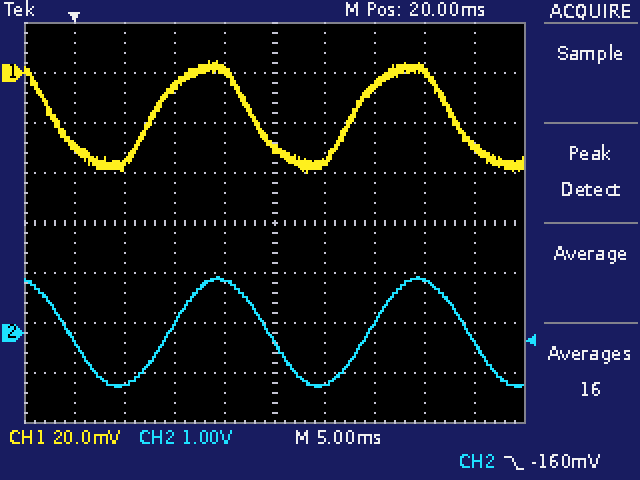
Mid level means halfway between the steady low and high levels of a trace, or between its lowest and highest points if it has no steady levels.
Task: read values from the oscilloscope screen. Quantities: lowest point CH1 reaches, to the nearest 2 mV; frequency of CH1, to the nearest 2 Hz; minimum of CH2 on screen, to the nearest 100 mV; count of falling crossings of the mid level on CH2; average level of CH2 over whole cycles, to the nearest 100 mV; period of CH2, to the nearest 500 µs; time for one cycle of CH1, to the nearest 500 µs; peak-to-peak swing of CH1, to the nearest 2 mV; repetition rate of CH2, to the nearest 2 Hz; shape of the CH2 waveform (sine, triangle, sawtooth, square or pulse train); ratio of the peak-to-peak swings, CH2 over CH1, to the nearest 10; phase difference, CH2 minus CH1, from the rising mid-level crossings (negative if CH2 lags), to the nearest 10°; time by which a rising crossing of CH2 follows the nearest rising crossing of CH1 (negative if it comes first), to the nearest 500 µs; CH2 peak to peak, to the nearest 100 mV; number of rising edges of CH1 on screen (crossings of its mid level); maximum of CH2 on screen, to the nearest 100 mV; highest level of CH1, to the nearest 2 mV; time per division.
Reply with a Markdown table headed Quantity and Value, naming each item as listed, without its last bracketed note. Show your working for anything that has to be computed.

| Quantity | Value |
|---|---|
| lowest point CH1 reaches, to the nearest 2 mV | -40 mV |
| frequency of CH1, to the nearest 2 Hz | 1 / 20.0 ms ≈ 50 Hz |
| minimum of CH2 on screen, to the nearest 100 mV | -1.1 V |
| count of falling crossings of the mid level on CH2 | 3 |
| average level of CH2 over whole cycles, to the nearest 100 mV | (1.1 V + (-1.1 V)) / 2 ≈ 0.0 V |
| period of CH2, to the nearest 500 µs | 20.0 ms |
| time for one cycle of CH1, to the nearest 500 µs | 20.0 ms |
| peak-to-peak swing of CH1, to the nearest 2 mV | 4 mV − (-40 mV) = 44 mV |
| repetition rate of CH2, to the nearest 2 Hz | 1 / 20.0 ms ≈ 50 Hz |
| shape of the CH2 waveform | sine |
| ratio of the peak-to-peak swings, CH2 over CH1, to the nearest 10 | 2.2 V / 44 mV ≈ 50 |
| phase difference, CH2 minus CH1, from the rising mid-level crossings (negative if CH2 lags), to the nearest 10° | −360° × (+1.5 ms) / 20.0 ms ≈ -27.0°, so -30° to the nearest 10° |
| time by which a rising crossing of CH2 follows the nearest rising crossing of CH1 (negative if it comes first), to the nearest 500 µs | +1.5 ms |
| CH2 peak to peak, to the nearest 100 mV | 1.1 V − (-1.1 V) = 2.2 V |
| number of rising edges of CH1 on screen | 2 |
| maximum of CH2 on screen, to the nearest 100 mV | 1.1 V |
| highest level of CH1, to the nearest 2 mV | 4 mV |
| time per division | 5 ms |
